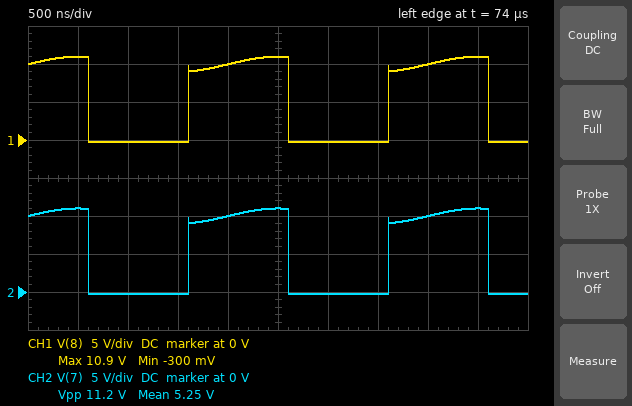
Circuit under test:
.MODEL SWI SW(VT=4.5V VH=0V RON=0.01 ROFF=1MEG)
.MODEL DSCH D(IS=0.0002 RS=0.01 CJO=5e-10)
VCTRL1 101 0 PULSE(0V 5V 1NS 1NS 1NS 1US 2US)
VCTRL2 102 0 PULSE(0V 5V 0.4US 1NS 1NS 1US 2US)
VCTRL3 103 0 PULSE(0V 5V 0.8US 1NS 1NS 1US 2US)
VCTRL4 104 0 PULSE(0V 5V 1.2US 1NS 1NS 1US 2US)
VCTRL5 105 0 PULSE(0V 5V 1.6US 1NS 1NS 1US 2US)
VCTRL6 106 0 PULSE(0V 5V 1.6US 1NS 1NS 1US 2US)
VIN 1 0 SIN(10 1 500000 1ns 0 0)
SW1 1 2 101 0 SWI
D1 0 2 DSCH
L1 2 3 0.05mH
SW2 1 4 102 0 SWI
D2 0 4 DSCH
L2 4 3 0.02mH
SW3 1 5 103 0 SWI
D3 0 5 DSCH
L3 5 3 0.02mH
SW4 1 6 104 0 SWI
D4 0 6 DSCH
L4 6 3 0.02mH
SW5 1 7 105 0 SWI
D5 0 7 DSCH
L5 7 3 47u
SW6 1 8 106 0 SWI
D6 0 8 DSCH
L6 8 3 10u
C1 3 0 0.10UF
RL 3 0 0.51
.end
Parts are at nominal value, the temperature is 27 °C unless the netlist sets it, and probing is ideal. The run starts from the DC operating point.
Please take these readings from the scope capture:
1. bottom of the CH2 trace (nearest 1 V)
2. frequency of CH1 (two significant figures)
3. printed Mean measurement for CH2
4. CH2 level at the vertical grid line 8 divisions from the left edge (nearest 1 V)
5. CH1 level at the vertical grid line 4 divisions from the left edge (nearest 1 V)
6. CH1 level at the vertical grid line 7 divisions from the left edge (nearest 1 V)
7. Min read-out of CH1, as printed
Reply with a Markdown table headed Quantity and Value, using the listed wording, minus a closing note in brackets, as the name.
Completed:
| Quantity | Value |
|---|---|
| bottom of the CH2 trace | 0 V |
| frequency of CH1 | 500 kHz |
| printed Mean measurement for CH2 | 5.25 V |
| CH2 level at the vertical grid line 8 divisions from the left edge | 10 V |
| CH1 level at the vertical grid line 4 divisions from the left edge | 10 V |
| CH1 level at the vertical grid line 7 divisions from the left edge | 0 V |
| Min read-out of CH1, as printed | -300 mV |
